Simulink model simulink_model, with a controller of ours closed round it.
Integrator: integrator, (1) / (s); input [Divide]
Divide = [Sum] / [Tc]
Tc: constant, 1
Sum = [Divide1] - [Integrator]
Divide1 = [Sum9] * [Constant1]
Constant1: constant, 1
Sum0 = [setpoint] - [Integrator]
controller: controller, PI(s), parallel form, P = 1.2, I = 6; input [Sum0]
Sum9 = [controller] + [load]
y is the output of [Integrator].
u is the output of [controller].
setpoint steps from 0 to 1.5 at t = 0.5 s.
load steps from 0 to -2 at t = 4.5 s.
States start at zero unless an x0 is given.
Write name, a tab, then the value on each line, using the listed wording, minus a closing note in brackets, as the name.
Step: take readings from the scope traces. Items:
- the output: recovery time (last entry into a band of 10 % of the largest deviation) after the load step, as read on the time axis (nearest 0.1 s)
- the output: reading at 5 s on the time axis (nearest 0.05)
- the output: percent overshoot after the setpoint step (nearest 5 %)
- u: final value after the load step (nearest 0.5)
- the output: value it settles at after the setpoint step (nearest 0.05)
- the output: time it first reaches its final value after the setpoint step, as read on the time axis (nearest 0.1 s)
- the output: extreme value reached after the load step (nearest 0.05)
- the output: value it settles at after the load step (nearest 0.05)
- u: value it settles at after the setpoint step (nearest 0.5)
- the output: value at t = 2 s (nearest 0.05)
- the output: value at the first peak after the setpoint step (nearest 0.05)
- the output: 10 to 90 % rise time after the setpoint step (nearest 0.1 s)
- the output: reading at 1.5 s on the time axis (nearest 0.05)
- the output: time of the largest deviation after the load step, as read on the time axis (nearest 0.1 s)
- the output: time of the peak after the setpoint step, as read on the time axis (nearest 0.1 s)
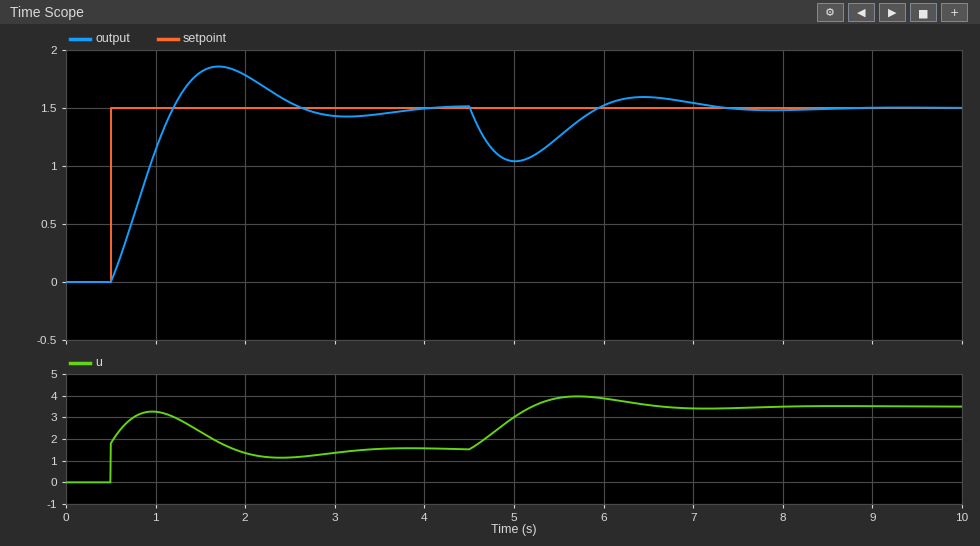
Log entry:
the output: recovery time (last entry into a band of 10 % of the largest deviation) after the load step, as read on the time axis	7.0 s
the output: reading at 5 s on the time axis	1.05
the output: percent overshoot after the setpoint step	25 %
u: final value after the load step	3.5
the output: value it settles at after the setpoint step	1.50
the output: time it first reaches its final value after the setpoint step, as read on the time axis	1.2 s
the output: extreme value reached after the load step	1.05
the output: value it settles at after the load step	1.50
u: value it settles at after the setpoint step	1.5
the output: value at t = 2 s	1.80
the output: value at the first peak after the setpoint step	1.85
the output: 10 to 90 % rise time after the setpoint step	0.5 s
the output: reading at 1.5 s on the time axis	1.80
the output: time of the largest deviation after the load step, as read on the time axis	5.0 s
the output: time of the peak after the setpoint step, as read on the time axis	1.7 s
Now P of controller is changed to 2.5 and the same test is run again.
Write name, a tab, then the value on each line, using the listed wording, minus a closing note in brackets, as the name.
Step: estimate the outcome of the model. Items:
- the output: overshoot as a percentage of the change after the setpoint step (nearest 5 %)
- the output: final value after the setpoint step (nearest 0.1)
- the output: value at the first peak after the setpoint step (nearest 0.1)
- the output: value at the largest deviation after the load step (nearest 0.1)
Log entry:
the output: overshoot as a percentage of the change after the setpoint step	10 %
the output: final value after the setpoint step	1.5
the output: value at the first peak after the setpoint step	1.7
the output: value at the largest deviation after the load step	1.1
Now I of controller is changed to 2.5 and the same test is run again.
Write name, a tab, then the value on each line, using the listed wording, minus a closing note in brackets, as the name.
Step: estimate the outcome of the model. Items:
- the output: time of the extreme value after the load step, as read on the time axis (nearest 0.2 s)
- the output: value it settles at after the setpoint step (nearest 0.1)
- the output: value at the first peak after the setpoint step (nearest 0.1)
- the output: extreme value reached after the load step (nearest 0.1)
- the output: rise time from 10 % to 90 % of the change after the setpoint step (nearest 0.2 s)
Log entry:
the output: time of the extreme value after the load step, as read on the time axis	5.2 s
the output: value it settles at after the setpoint step	1.5
the output: value at the first peak after the setpoint step	1.6
the output: extreme value reached after the load step	0.9
the output: rise time from 10 % to 90 % of the change after the setpoint step	1.0 s
